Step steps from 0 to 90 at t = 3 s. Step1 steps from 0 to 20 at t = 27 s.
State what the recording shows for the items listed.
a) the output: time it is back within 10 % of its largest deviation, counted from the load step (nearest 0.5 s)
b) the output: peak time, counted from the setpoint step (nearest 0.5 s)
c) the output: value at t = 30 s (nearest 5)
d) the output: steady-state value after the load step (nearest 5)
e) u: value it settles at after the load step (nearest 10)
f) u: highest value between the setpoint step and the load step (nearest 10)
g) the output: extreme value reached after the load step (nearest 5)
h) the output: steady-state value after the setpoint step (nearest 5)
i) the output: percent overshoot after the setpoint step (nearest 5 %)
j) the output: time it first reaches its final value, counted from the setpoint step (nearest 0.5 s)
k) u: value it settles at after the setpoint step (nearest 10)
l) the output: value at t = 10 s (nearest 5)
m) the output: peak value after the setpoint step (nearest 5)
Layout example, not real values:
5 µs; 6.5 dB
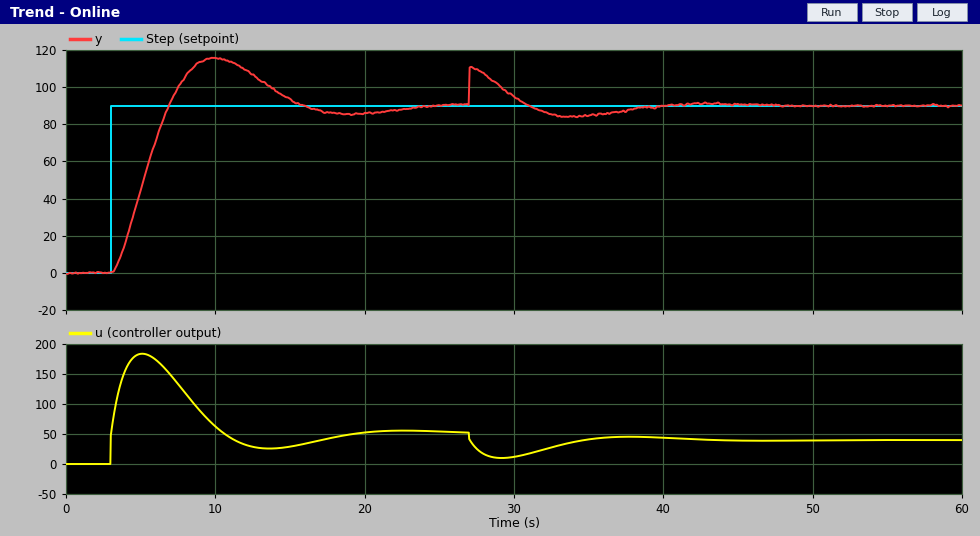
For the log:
11.0 s; 7.0 s; 95; 90; 40; 180; 110; 90; 30 %; 4.0 s; 50; 115; 115
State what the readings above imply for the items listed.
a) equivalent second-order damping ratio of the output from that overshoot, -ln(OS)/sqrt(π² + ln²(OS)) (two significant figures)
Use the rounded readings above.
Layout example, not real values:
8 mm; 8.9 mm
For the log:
0.36
